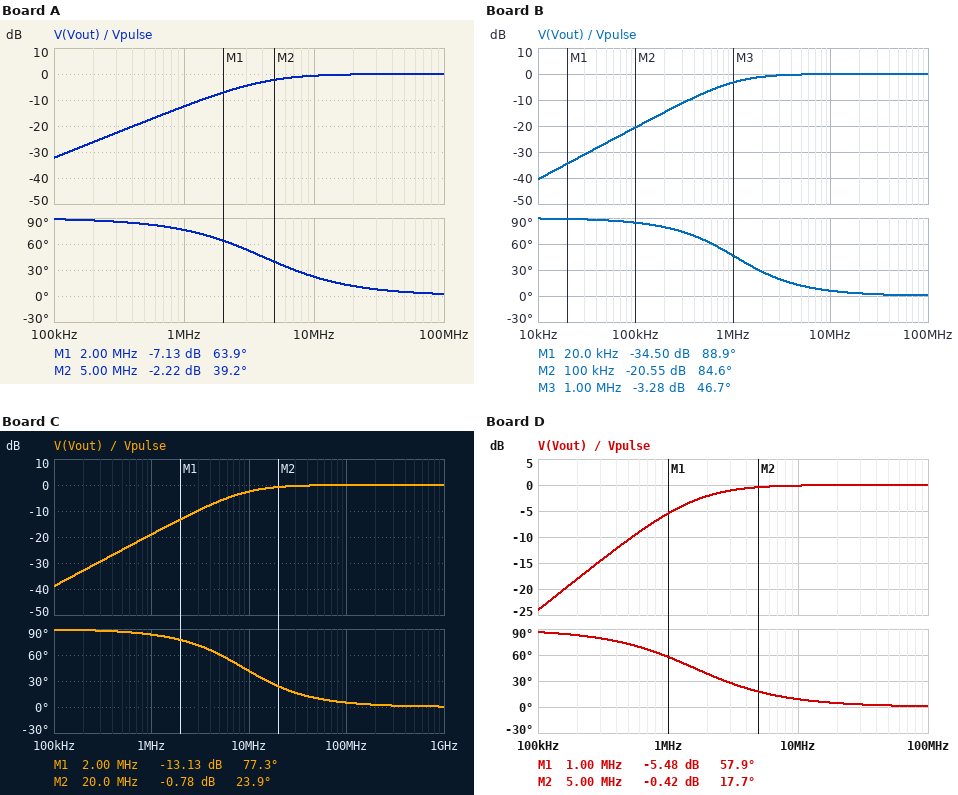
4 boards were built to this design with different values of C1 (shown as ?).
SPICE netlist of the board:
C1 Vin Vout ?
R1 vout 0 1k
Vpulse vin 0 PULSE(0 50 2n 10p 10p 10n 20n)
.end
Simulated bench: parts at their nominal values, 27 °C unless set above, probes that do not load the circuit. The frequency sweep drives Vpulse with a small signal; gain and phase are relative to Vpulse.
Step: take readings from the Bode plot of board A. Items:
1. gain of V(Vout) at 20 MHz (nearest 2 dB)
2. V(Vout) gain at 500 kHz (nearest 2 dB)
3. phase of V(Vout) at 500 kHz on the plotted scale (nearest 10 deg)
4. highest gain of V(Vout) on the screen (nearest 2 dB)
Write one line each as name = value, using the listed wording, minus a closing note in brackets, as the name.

gain of V(Vout) at 20 MHz = 0 dB
V(Vout) gain at 500 kHz = -18 dB
phase of V(Vout) at 500 kHz on the plotted scale = 80 deg
highest gain of V(Vout) on the screen = 0 dB
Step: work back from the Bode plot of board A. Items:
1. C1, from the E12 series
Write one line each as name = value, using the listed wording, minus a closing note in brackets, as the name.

C1, from the E12 series = 39 pF
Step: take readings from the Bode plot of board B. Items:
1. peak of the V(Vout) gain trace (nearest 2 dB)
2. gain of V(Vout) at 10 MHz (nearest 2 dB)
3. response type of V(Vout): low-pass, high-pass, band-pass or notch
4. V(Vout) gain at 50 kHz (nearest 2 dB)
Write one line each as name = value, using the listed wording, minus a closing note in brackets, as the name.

peak of the V(Vout) gain trace = 0 dB
gain of V(Vout) at 10 MHz = 0 dB
response type of V(Vout): low-pass, high-pass, band-pass or notch = high-pass
V(Vout) gain at 50 kHz = -26 dB
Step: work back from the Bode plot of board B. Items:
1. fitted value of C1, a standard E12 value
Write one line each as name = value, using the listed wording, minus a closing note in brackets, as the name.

fitted value of C1, a standard E12 value = 150 pF
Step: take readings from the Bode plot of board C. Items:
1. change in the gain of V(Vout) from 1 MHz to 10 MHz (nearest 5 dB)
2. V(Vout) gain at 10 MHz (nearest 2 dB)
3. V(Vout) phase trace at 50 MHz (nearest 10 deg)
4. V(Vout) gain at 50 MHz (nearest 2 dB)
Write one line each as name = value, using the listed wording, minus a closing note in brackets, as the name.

change in the gain of V(Vout) from 1 MHz to 10 MHz = 15 dB
V(Vout) gain at 10 MHz = -2 dB
V(Vout) phase trace at 50 MHz = 10 deg
V(Vout) gain at 50 MHz = 0 dB
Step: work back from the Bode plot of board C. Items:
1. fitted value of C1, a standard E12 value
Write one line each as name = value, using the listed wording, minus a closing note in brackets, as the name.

fitted value of C1, a standard E12 value = 18 pF
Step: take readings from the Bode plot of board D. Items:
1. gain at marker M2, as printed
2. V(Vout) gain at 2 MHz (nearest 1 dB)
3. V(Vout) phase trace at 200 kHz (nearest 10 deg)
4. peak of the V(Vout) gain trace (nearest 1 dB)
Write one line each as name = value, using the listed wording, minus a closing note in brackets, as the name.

gain at marker M2, as printed = -0.42 dB
V(Vout) gain at 2 MHz = -2 dB
V(Vout) phase trace at 200 kHz = 80 deg
peak of the V(Vout) gain trace = 0 dB
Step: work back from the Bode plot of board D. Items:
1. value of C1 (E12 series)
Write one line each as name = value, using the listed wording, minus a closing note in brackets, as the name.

value of C1 = 100 pF
